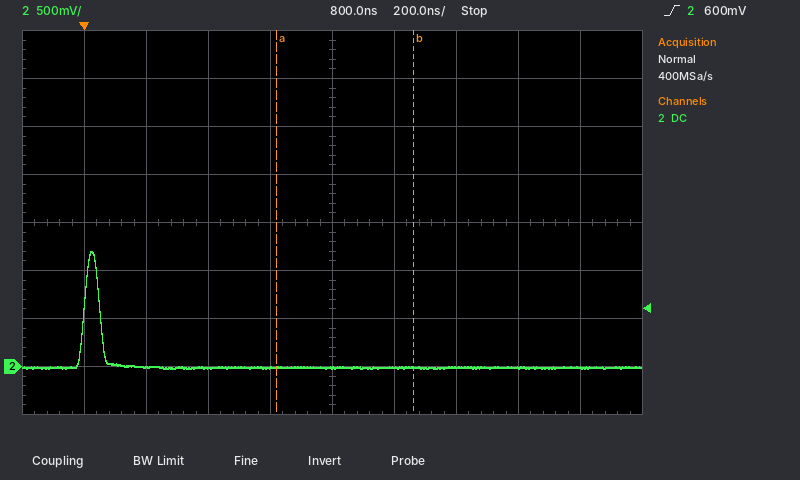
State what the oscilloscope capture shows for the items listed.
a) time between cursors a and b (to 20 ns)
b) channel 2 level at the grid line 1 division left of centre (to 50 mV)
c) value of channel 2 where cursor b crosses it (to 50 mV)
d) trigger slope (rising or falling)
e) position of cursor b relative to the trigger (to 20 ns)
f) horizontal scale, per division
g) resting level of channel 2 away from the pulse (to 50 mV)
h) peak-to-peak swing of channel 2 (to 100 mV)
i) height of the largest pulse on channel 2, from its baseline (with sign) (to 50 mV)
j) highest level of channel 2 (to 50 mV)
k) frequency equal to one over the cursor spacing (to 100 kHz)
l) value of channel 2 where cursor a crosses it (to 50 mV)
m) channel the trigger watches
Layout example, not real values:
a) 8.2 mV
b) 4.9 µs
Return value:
a) 440 ns
b) 0 mV
c) 0 mV
d) rising
e) +1.06 µs
f) 200 ns
g) 0 mV
h) 1.20 V
i) +1.20 V
j) 1.20 V
k) 2.3 MHz
l) 0 mV
m) channel 2
